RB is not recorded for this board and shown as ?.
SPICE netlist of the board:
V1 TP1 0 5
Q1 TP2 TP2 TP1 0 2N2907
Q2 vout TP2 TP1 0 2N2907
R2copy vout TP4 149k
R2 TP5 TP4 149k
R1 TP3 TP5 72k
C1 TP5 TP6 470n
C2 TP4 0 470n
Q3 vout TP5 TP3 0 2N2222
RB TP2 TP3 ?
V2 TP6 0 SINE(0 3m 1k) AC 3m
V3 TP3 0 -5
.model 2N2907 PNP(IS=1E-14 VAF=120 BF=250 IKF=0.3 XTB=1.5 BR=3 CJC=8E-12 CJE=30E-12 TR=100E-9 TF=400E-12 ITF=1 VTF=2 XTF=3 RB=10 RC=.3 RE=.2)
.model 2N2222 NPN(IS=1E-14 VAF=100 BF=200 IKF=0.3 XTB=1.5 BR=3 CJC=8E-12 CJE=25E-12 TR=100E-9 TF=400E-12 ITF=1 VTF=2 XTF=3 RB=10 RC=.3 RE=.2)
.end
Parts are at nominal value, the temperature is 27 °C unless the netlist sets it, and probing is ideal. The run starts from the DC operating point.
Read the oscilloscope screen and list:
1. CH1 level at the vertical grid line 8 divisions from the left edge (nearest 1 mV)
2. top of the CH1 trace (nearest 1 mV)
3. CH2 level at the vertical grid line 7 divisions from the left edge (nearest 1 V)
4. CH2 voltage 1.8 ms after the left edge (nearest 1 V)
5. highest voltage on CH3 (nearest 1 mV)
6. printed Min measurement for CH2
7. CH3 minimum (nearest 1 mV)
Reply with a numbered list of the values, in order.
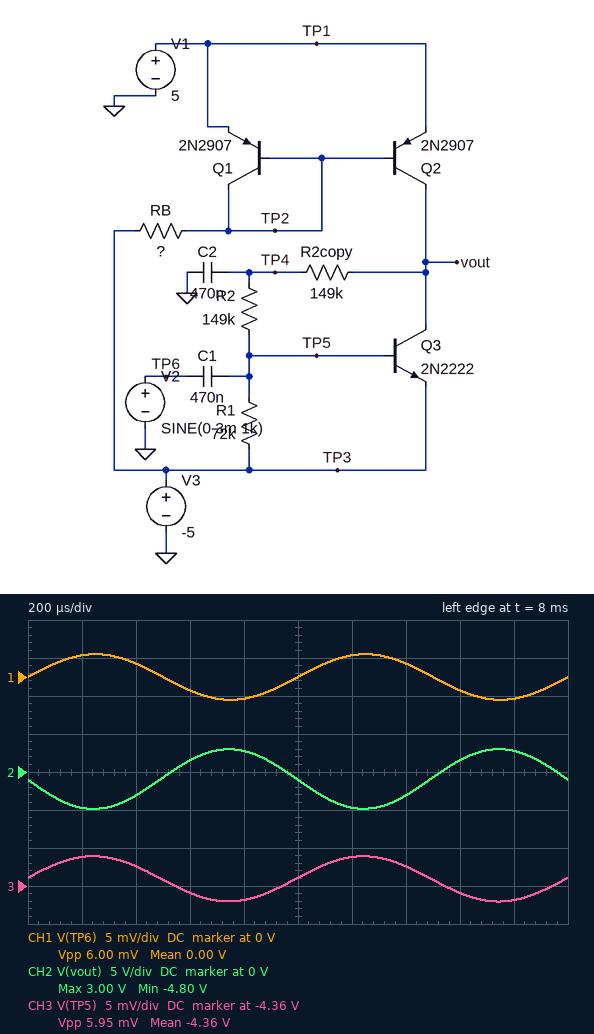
1. -2 mV
2. 3 mV
3. -3 V
4. 3 V
5. -4.356 V
6. -4.80 V
7. -4.362 V
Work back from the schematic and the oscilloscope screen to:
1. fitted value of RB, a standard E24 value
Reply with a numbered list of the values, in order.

1. 16 kΩ
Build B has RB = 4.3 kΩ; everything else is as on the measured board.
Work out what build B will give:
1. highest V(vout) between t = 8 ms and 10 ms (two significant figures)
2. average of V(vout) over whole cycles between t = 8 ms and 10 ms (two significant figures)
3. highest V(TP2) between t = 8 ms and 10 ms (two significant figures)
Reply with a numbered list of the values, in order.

1. 4.9 V
2. 1.5 V
3. 4.3 V
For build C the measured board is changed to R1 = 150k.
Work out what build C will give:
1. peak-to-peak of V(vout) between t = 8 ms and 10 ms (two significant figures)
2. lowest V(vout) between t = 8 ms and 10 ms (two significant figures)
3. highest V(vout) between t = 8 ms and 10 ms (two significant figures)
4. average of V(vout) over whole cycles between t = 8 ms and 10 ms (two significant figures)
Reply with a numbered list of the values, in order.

1. 6.9 V
2. -4.9 V
3. 2.0 V
4. -1.7 V
